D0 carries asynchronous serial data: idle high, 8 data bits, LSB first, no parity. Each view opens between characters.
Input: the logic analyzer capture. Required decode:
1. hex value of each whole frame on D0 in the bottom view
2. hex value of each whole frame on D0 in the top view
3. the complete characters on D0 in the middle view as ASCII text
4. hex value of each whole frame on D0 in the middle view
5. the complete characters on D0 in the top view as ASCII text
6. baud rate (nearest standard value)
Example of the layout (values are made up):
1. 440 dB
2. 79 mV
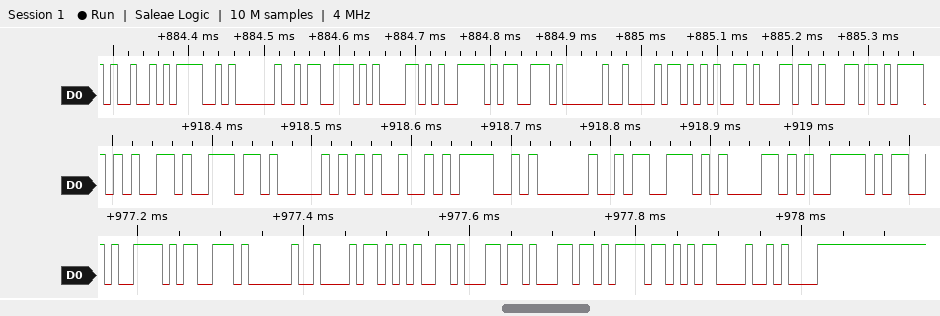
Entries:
1. 79, 73, 20, 68, 65, 6C, 6C, 6F, 0D, 0A
2. 49, 4F, 20, 73, 61, 79, 73, 20, 68, 65, 6C, 6C
3. "enPIO say"
4. 65, 6E, 50, 49, 4F, 20, 73, 61, 79
5. "IO says hell"
6. 115200 baud
